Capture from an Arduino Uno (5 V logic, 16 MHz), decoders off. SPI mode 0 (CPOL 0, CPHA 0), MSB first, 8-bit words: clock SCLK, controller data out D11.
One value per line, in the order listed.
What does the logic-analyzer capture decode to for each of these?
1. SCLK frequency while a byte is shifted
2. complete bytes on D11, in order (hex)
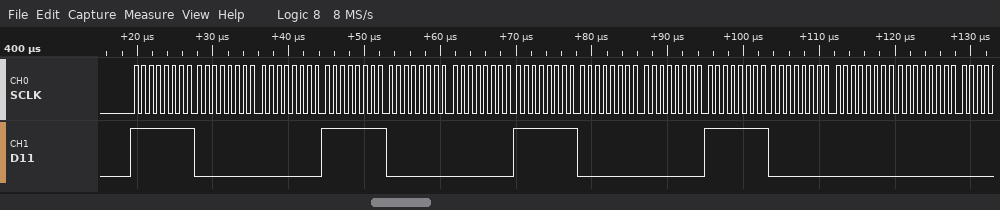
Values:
1 MHz
FF 00 00 FF 00 00 FF 00 00 FF 00 00 00
